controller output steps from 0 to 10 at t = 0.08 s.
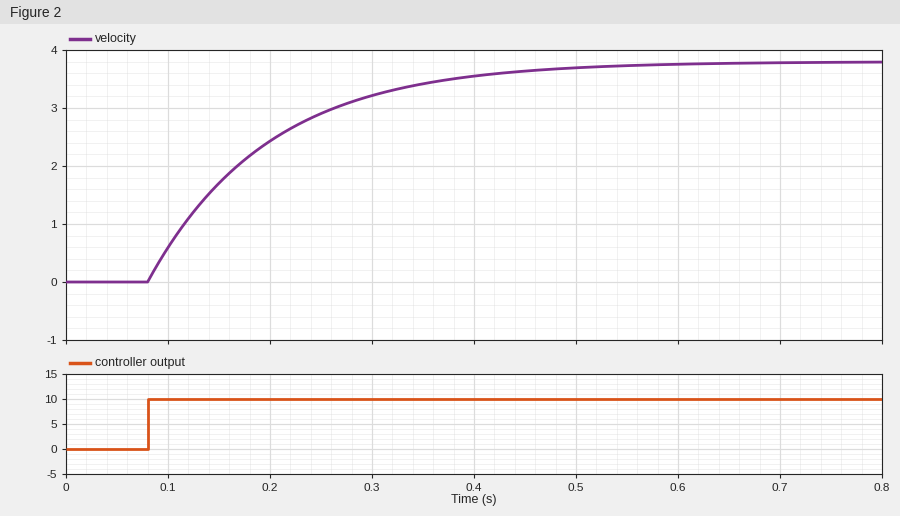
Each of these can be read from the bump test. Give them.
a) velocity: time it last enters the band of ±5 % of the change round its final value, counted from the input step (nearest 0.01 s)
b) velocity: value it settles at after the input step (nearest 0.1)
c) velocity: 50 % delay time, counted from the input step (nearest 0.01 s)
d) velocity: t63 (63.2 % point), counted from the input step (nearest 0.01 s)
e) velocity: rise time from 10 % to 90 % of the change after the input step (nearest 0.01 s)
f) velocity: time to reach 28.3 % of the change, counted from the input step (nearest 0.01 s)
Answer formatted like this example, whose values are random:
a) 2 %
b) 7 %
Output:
a) 0.35 s
b) 3.8
c) 0.08 s
d) 0.12 s
e) 0.26 s
f) 0.04 s
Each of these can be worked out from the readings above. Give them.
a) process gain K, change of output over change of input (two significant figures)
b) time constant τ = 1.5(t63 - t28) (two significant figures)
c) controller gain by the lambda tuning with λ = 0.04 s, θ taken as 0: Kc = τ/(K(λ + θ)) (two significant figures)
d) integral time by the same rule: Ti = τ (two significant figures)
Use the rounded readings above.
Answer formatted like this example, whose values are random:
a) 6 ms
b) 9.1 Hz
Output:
a) 0.38
b) 0.12 s
c) 7.9
d) 0.12 s
